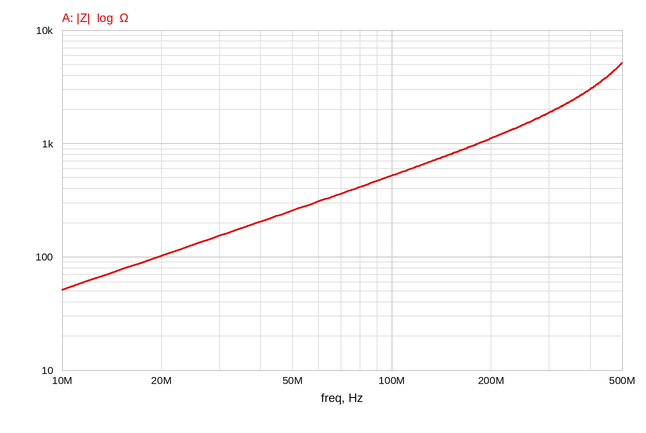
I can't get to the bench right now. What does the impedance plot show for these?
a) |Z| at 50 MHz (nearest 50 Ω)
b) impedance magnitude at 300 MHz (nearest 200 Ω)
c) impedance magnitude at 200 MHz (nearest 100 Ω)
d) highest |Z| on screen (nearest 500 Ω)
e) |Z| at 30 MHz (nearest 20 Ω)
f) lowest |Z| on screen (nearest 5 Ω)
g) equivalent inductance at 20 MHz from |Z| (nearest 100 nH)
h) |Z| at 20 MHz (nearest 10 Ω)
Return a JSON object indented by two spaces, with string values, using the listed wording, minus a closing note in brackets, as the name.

{
  "|Z| at 50 MHz": "250 Ω",
  "impedance magnitude at 300 MHz": "1.8 kΩ",
  "impedance magnitude at 200 MHz": "1.1 kΩ",
  "highest |Z| on screen": "5.0 kΩ",
  "|Z| at 30 MHz": "160 Ω",
  "lowest |Z| on screen": "50 Ω",
  "equivalent inductance at 20 MHz from |Z|": "800 nH",
  "|Z| at 20 MHz": "100 Ω"
}
